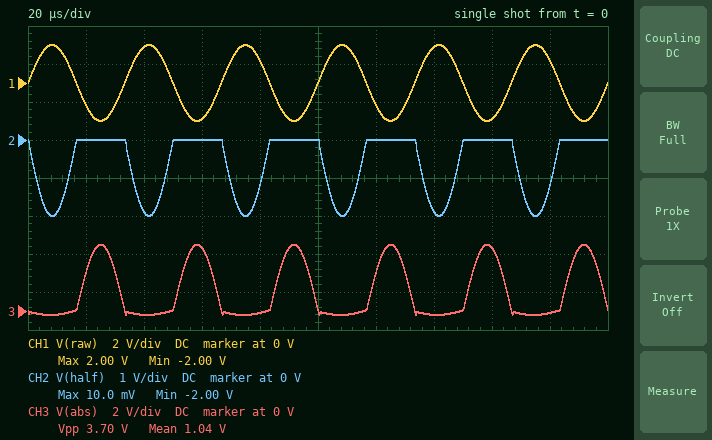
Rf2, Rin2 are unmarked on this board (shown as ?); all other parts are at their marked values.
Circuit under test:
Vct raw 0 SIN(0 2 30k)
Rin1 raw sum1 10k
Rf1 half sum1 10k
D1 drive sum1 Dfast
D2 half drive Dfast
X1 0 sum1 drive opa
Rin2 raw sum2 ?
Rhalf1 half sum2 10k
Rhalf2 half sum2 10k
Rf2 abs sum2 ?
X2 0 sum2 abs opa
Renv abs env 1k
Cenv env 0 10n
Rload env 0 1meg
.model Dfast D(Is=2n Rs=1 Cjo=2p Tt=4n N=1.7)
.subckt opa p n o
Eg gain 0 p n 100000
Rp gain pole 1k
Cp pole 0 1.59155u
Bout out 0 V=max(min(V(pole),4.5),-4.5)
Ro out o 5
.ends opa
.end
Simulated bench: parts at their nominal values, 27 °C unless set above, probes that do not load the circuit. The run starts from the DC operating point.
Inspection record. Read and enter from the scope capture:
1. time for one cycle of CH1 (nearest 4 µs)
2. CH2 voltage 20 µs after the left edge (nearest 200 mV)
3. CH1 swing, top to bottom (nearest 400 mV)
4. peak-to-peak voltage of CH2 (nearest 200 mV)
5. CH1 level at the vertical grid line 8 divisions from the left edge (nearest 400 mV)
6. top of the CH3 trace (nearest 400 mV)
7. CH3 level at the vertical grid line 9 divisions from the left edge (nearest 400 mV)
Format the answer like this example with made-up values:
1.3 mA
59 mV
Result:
32 µs
0 V
4.0 V
2.0 V
-2.0 V
3.6 V
0 V
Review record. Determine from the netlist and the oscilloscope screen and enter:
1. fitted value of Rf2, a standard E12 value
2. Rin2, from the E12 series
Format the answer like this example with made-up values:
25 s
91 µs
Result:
8.2 kΩ
4.7 kΩ
